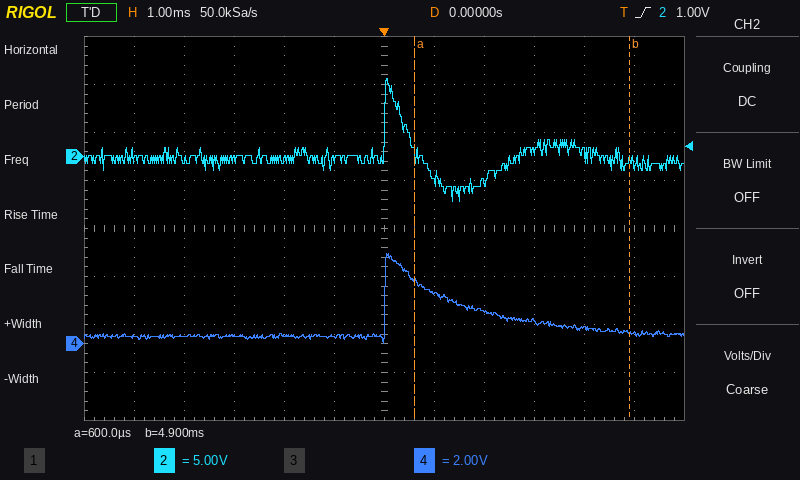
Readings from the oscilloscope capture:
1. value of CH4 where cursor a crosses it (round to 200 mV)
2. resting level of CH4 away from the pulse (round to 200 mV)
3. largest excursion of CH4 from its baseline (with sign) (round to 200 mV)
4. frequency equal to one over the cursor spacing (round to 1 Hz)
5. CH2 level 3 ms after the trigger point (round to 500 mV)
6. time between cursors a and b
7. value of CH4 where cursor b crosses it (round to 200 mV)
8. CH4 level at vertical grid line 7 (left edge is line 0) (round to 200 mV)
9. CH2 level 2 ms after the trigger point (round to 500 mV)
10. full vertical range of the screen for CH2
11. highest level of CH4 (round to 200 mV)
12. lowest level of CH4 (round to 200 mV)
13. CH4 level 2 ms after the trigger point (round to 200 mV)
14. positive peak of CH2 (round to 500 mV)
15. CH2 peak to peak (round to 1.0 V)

2.6 V
400 mV
+3.4 V
233 Hz
500 mV
4.3 ms
400 mV
2.2 V
-2.5 V
40 V
3.8 V
0.0 V
1.4 V
8.0 V
13.0 V
